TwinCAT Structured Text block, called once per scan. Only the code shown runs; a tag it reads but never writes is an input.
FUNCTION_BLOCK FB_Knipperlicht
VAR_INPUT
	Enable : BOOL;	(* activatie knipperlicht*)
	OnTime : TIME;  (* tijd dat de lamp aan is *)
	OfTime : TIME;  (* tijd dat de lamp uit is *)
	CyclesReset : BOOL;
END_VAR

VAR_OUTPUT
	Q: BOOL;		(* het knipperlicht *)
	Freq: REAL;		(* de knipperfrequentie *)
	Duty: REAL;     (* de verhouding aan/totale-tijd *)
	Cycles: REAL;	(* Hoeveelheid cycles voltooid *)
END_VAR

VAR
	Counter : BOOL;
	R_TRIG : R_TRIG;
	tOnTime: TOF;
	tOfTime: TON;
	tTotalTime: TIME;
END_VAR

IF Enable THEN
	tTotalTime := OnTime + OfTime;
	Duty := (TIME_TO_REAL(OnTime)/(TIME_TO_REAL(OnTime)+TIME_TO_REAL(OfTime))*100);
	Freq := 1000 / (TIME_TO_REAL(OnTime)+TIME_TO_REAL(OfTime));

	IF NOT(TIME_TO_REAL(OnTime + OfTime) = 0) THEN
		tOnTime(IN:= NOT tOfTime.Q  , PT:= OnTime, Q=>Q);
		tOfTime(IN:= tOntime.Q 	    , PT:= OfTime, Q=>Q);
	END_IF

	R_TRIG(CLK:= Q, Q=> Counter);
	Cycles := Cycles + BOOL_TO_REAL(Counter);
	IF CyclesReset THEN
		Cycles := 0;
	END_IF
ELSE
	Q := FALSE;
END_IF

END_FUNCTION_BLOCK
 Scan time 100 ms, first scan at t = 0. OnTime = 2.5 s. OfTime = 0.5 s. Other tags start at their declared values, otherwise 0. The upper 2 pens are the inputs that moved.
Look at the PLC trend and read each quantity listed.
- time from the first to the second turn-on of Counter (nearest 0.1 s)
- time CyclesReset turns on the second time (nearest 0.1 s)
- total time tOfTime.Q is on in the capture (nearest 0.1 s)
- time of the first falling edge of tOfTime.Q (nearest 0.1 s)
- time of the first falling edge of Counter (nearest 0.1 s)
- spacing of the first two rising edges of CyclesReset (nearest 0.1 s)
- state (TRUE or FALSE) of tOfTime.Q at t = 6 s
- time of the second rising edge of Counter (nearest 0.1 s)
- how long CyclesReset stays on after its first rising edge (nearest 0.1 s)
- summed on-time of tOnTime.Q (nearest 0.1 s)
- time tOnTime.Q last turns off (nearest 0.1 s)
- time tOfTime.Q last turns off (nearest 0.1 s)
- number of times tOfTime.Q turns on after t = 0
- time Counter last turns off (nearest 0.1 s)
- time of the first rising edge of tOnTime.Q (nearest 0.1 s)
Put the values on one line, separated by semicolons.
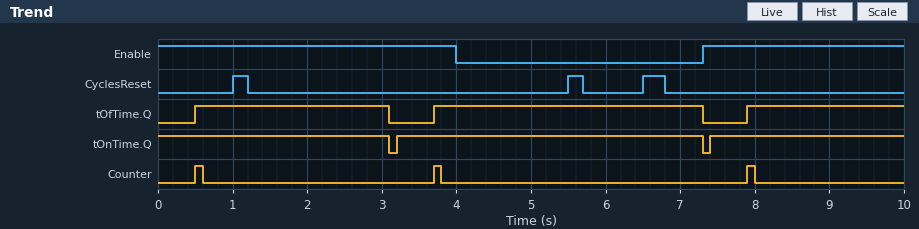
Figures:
3.2 s; 5.5 s; 8.3 s; 3.1 s; 0.6 s; 4.5 s; TRUE; 3.7 s; 0.2 s; 9.8 s; 7.3 s; 7.3 s; 3; 8.0 s; 3.2 s
